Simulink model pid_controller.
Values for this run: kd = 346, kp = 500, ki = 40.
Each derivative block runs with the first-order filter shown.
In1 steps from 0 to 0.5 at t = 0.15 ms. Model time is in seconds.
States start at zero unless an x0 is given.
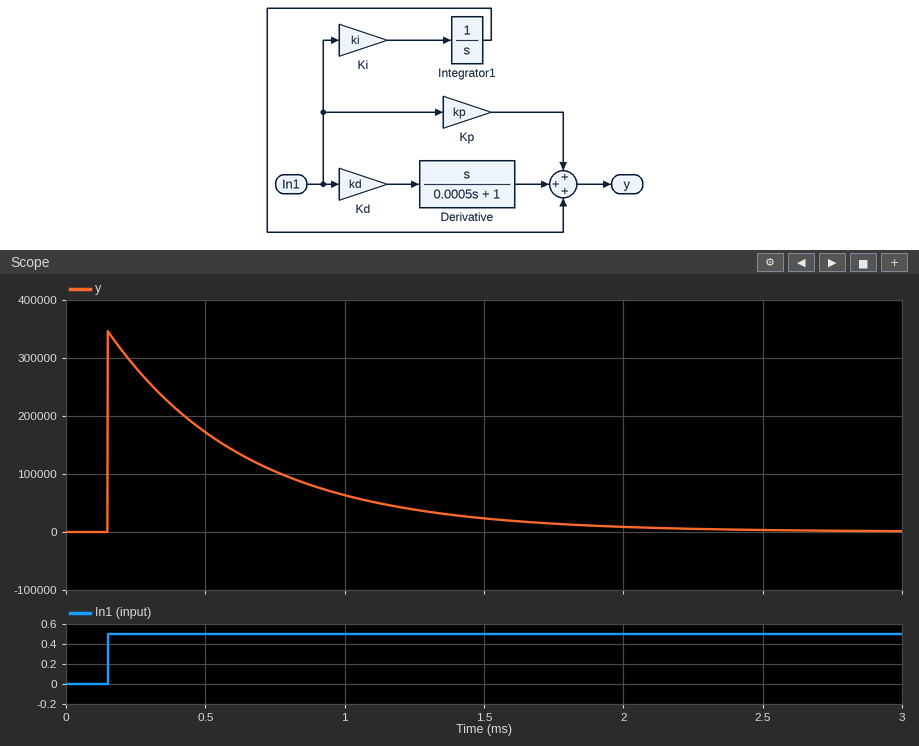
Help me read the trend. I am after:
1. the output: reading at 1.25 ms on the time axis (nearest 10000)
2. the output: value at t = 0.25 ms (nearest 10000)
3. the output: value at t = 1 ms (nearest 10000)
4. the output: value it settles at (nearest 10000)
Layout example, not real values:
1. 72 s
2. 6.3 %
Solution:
1. 40000
2. 280000
3. 60000
4. 0
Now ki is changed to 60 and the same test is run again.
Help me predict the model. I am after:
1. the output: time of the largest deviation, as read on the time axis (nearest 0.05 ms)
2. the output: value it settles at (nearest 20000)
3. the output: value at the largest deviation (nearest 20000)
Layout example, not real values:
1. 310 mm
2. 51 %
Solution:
1. 0.15 ms
2. 0
3. 340000
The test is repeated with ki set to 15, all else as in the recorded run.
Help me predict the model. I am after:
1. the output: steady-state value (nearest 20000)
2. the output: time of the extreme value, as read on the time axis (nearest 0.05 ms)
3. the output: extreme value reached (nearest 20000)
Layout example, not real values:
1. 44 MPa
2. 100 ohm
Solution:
1. 0
2. 0.15 ms
3. 340000
